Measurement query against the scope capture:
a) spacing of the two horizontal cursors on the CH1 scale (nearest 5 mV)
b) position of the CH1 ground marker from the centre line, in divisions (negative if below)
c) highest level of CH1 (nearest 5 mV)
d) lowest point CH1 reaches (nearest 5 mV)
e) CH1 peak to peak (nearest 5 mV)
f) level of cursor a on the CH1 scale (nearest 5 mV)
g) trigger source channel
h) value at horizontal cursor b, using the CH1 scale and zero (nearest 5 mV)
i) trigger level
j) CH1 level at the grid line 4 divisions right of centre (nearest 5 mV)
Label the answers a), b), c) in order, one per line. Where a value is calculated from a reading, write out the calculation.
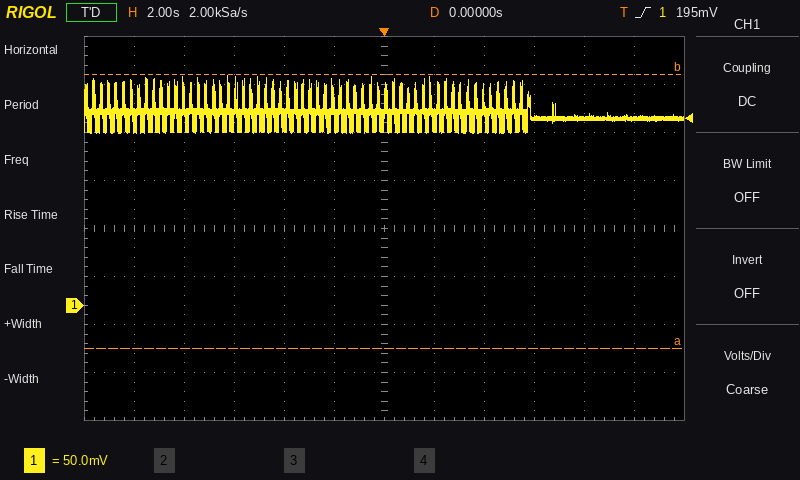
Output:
a) 285 mV
b) -1.6 div
c) 240 mV
d) 180 mV
e) 240 mV − (180 mV) = 60 mV
f) -45 mV
g) CH1
h) 240 mV
i) 195 mV
j) 195 mV
